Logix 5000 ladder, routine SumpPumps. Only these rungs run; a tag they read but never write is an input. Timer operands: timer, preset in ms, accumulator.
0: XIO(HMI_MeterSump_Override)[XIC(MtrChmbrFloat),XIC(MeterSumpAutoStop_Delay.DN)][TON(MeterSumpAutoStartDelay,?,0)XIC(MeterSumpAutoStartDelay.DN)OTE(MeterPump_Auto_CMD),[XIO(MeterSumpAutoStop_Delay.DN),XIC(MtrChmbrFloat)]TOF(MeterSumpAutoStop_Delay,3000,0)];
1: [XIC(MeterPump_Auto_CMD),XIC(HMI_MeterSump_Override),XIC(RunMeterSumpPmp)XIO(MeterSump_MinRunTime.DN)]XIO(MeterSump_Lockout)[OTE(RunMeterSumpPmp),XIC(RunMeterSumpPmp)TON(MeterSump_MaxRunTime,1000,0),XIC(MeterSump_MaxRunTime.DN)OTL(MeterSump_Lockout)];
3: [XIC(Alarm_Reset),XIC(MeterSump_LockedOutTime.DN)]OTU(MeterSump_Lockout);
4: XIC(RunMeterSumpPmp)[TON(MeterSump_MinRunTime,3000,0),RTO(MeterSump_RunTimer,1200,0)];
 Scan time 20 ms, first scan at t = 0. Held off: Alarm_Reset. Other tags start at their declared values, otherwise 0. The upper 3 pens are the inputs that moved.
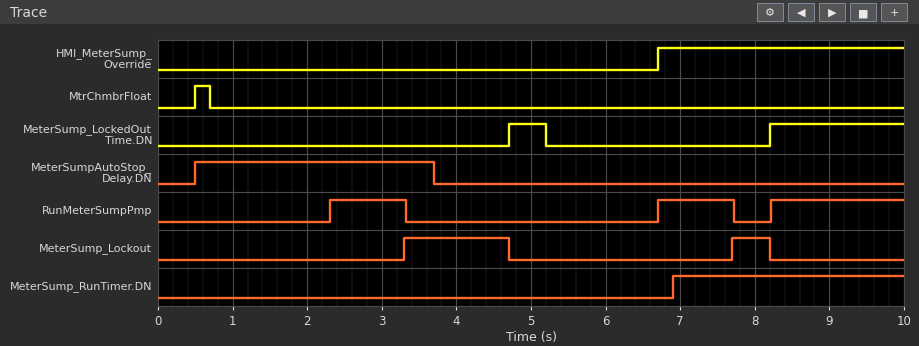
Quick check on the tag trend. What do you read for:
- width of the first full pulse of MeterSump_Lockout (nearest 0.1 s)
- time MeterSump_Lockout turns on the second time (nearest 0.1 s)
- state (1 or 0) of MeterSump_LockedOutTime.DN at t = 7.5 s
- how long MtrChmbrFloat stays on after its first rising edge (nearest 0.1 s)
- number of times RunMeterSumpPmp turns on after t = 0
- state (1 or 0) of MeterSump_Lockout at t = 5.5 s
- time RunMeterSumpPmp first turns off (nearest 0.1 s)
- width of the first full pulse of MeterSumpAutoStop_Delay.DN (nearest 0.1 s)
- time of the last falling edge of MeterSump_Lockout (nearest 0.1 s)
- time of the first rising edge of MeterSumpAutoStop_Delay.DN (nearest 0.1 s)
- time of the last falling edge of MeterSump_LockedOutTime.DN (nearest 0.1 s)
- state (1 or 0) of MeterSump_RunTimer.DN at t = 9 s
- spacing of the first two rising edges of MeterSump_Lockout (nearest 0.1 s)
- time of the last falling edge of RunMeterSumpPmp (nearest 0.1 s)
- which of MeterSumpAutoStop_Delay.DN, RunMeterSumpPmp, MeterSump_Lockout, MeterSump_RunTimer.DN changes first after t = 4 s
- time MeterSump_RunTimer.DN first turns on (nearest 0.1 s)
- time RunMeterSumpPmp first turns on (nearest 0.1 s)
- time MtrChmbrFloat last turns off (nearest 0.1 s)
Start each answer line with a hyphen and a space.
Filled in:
- 1.4 s
- 7.7 s
- 0
- 0.2 s
- 3
- 0
- 3.3 s
- 3.2 s
- 8.2 s
- 0.5 s
- 5.2 s
- 1
- 4.4 s
- 7.7 s
- MeterSump_Lockout
- 6.9 s
- 2.3 s
- 0.7 s
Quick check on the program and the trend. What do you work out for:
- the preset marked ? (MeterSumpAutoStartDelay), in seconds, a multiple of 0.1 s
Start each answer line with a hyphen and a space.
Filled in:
- 1.8 s
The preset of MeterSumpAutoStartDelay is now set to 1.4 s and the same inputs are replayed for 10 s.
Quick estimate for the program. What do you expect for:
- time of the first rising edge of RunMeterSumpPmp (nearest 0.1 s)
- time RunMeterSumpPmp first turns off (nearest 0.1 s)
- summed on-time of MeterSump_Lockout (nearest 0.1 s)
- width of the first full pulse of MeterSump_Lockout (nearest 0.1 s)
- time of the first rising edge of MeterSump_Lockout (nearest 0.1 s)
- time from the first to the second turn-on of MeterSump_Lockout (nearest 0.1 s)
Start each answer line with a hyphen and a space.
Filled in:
- 1.9 s
- 2.9 s
- 2.3 s
- 1.8 s
- 2.9 s
- 4.8 s
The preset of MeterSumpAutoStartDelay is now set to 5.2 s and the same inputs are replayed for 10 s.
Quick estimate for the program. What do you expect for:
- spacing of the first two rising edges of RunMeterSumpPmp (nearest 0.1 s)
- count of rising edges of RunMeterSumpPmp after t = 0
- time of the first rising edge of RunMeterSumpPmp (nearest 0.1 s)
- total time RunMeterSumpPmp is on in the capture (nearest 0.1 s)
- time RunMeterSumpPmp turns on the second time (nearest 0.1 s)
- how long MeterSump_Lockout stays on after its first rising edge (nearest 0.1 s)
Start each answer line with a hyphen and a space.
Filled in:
- 1.5 s
- 2
- 6.7 s
- 2.8 s
- 8.2 s
- 0.5 s
